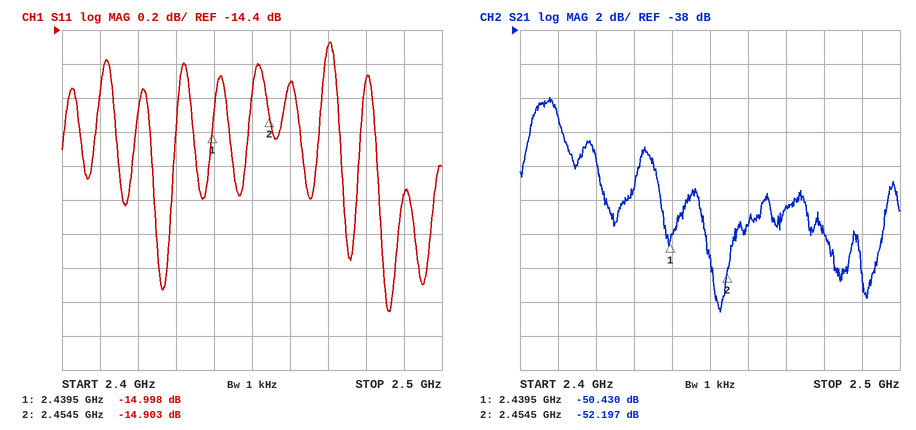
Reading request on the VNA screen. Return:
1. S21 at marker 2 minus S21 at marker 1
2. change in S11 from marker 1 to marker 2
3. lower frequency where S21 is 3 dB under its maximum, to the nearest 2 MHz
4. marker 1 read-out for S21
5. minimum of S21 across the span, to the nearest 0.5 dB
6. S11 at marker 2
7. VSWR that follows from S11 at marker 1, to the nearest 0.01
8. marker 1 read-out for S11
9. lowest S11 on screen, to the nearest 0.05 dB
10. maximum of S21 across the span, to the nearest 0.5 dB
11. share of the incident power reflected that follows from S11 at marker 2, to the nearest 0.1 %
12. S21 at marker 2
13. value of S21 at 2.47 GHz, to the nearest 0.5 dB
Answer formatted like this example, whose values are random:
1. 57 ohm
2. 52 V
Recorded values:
1. -1.767 dB
2. 0.095 dB
3. 2.402 GHz
4. -50.430 dB
5. -54.5 dB
6. -14.903 dB
7. 1.43
8. -14.998 dB
9. -16.05 dB
10. -42.0 dB
11. 3.2 %
12. -52.197 dB
13. -48.5 dB
